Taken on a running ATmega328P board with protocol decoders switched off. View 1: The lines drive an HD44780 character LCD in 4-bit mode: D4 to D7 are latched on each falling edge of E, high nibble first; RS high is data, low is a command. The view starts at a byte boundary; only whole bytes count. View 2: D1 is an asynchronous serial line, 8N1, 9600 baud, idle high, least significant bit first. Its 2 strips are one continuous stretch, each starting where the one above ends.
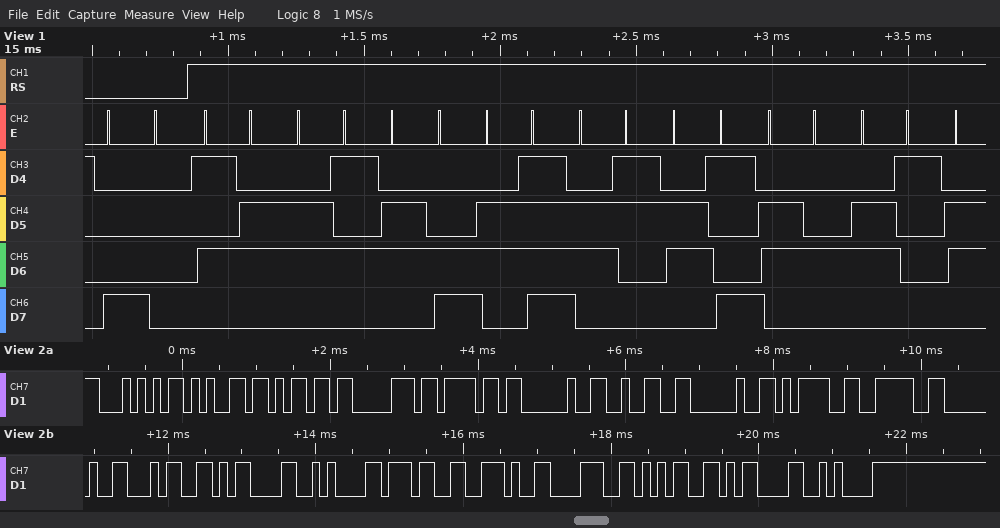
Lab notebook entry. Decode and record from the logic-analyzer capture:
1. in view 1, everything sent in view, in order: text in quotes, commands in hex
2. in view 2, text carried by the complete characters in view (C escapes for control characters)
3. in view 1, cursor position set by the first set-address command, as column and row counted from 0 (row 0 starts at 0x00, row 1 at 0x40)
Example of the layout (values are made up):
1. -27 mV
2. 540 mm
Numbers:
1. 0x80 "Velocida"
2. "Tempo 2 => 4\r\n7.85\r\n"
3. column 0, row 0
